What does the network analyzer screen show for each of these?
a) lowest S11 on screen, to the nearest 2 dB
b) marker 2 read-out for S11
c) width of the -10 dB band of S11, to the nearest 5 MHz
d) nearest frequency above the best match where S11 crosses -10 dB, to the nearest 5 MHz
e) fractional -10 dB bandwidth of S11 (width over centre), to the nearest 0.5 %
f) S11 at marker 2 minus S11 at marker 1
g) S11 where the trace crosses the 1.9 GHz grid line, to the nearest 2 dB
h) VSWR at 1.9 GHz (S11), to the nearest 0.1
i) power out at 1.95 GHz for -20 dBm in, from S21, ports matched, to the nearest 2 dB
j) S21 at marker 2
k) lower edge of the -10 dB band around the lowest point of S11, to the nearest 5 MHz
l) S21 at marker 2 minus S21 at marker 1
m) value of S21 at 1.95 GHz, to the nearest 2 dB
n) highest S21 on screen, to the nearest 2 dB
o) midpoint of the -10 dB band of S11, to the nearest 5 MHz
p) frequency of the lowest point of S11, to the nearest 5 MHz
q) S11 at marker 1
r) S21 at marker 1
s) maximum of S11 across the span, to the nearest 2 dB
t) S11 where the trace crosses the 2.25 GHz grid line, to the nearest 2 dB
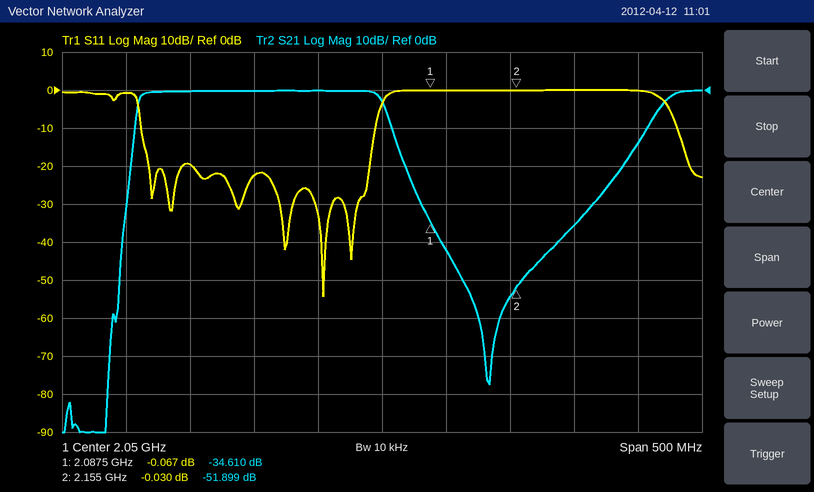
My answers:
-54 dB
-0.030 dB
185 MHz
2.045 GHz
9.5 %
0.037 dB
-20 dB
1.2
-20 dBm
-51.899 dB
1.860 GHz
-17.289 dB
0 dB
0 dB
1.955 GHz
2.005 GHz
-0.067 dB
-34.610 dB
0 dB
0 dB
